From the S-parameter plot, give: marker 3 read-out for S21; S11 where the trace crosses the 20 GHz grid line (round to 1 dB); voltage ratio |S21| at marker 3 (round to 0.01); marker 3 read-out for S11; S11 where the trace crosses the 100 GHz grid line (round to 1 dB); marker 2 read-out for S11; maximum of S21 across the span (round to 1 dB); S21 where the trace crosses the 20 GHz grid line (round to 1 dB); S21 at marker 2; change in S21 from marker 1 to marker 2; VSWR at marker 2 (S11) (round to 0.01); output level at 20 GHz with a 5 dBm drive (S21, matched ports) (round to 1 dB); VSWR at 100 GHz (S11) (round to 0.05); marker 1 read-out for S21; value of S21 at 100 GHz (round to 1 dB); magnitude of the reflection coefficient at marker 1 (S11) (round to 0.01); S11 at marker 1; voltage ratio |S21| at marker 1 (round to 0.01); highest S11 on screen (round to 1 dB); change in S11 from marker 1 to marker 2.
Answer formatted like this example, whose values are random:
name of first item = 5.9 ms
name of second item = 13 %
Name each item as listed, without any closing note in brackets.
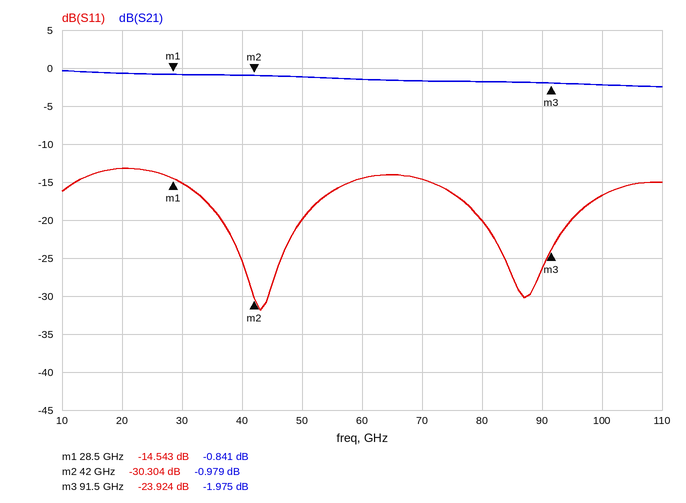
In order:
marker 3 read-out for S21 = -1.975 dB
S11 where the trace crosses the 20 GHz grid line = -13 dB
voltage ratio |S21| at marker 3 = 0.80
marker 3 read-out for S11 = -23.924 dB
S11 where the trace crosses the 100 GHz grid line = -17 dB
marker 2 read-out for S11 = -30.304 dB
maximum of S21 across the span = 0 dB
S21 where the trace crosses the 20 GHz grid line = -1 dB
S21 at marker 2 = -0.979 dB
change in S21 from marker 1 to marker 2 = -0.138 dB
VSWR at marker 2 (S11) = 1.06
output level at 20 GHz with a 5 dBm drive (S21, matched ports) = 4 dBm
VSWR at 100 GHz (S11) = 1.35
marker 1 read-out for S21 = -0.841 dB
value of S21 at 100 GHz = -2 dB
magnitude of the reflection coefficient at marker 1 (S11) = 0.19
S11 at marker 1 = -14.543 dB
voltage ratio |S21| at marker 1 = 0.91
highest S11 on screen = -13 dB
change in S11 from marker 1 to marker 2 = -15.761 dB
